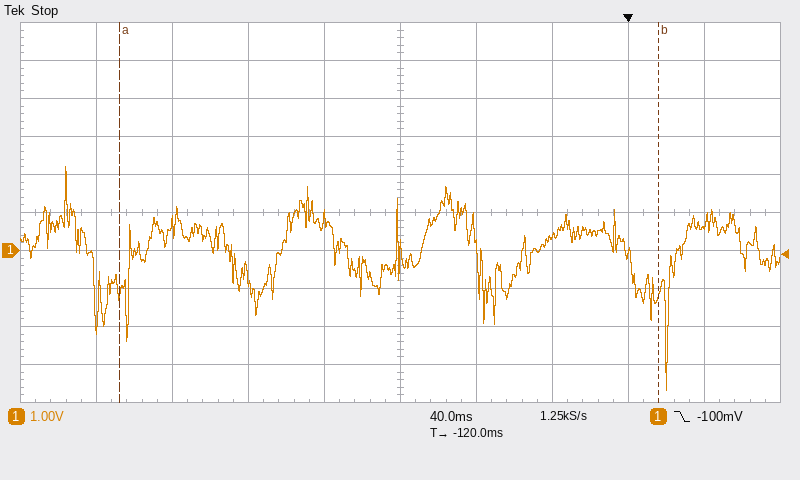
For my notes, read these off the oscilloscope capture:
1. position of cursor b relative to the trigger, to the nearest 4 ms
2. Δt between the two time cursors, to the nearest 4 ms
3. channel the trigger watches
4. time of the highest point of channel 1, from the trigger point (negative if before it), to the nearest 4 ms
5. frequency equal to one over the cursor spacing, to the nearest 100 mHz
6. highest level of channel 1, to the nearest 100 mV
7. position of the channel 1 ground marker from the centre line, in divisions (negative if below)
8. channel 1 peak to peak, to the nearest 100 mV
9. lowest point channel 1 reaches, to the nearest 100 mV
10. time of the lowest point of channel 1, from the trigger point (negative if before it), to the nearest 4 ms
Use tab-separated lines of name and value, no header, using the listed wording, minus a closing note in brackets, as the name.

position of cursor b relative to the trigger, to the nearest 4 ms	+16 ms
Δt between the two time cursors, to the nearest 4 ms	284 ms
channel the trigger watches	channel 1
time of the highest point of channel 1, from the trigger point (negative if before it), to the nearest 4 ms	-296 ms
frequency equal to one over the cursor spacing, to the nearest 100 mHz	3.5 Hz
highest level of channel 1, to the nearest 100 mV	2.2 V
position of the channel 1 ground marker from the centre line, in divisions	-1.0 div
channel 1 peak to peak, to the nearest 100 mV	5.9 V
lowest point channel 1 reaches, to the nearest 100 mV	-3.7 V
time of the lowest point of channel 1, from the trigger point (negative if before it), to the nearest 4 ms	+20 ms
